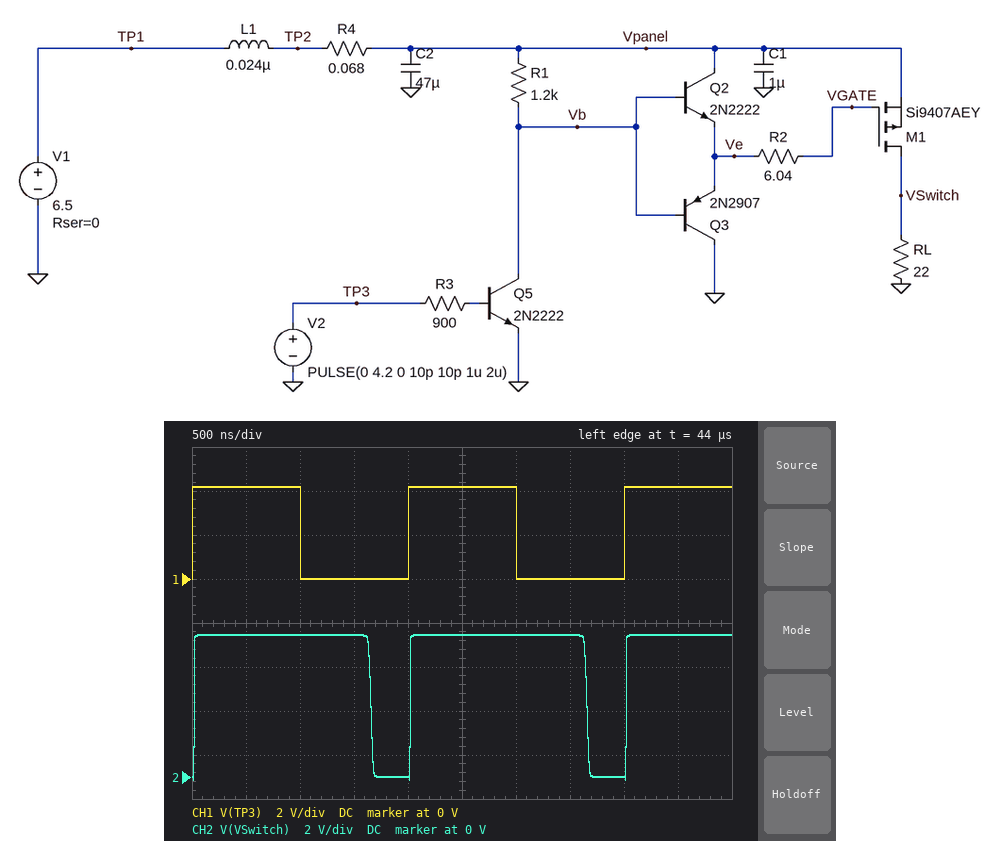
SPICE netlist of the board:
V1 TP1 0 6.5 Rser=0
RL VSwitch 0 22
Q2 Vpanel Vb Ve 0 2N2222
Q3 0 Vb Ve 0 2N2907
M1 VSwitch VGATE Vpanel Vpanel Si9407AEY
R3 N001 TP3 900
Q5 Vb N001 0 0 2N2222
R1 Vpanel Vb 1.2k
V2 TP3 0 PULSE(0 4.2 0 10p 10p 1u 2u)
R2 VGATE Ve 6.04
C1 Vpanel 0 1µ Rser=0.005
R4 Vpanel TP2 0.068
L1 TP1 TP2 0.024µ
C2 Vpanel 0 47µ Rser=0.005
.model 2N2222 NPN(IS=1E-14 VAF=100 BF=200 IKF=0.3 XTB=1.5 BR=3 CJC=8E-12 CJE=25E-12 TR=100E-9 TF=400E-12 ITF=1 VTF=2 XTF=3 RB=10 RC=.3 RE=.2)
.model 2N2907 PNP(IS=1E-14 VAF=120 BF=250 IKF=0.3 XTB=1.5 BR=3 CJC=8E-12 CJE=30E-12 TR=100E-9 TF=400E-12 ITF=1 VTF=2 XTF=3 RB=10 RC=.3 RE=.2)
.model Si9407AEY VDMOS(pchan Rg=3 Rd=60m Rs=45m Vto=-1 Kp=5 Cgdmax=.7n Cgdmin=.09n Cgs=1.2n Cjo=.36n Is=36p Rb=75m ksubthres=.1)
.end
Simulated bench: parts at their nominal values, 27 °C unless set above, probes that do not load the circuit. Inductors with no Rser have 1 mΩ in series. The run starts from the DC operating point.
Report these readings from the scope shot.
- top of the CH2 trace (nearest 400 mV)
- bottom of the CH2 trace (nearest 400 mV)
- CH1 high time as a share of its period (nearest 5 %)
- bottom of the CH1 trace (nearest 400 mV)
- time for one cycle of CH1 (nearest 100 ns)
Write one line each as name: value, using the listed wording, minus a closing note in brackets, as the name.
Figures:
top of the CH2 trace: 6.4 V
bottom of the CH2 trace: 0 V
CH1 high time as a share of its period: 50 %
bottom of the CH1 trace: 0 V
time for one cycle of CH1: 2.0 µs
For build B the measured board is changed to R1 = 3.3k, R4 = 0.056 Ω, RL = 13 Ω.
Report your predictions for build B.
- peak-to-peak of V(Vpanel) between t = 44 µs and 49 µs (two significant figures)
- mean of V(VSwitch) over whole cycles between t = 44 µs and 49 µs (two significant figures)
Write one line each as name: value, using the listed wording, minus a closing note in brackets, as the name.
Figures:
peak-to-peak of V(Vpanel) between t = 44 µs and 49 µs: 4.0 mV
mean of V(VSwitch) over whole cycles between t = 44 µs and 49 µs: 5.7 V
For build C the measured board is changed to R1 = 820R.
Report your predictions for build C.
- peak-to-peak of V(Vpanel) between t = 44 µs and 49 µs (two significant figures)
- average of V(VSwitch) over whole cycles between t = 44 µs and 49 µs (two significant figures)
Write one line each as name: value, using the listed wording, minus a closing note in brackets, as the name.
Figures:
peak-to-peak of V(Vpanel) between t = 44 µs and 49 µs: 3.2 mV
average of V(VSwitch) over whole cycles between t = 44 µs and 49 µs: 5.2 V
